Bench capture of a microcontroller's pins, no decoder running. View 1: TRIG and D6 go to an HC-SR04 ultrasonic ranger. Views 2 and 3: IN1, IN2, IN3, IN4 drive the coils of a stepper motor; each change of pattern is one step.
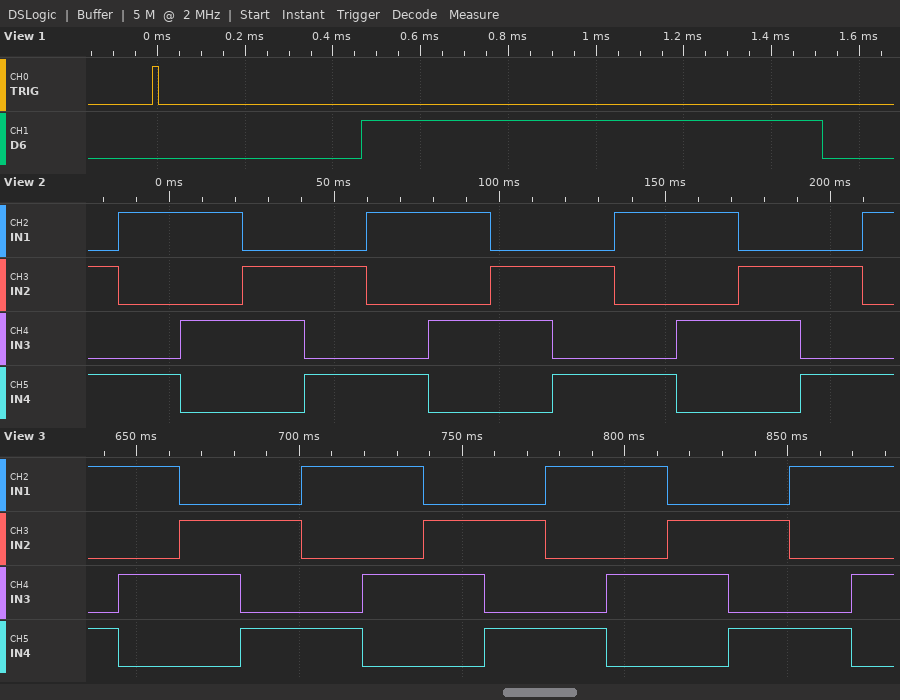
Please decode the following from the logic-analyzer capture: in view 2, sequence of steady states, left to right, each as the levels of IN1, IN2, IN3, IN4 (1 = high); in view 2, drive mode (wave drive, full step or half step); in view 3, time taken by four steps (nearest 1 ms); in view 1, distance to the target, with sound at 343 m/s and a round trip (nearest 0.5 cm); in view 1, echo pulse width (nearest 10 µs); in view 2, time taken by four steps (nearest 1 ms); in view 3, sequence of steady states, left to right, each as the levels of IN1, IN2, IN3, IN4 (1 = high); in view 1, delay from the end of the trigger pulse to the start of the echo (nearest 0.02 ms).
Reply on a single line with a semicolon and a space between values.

0101 1001 1010 0110 0101 1001 1010 0110 0101 1001 1010 0110 0101 1001; full step; 75 ms; 18 cm; 1050 µs; 75 ms; 1001 1010 0110 0101 1001 1010 0110 0101 1001 1010 0110 0101 1001 1010; 0.46 ms
